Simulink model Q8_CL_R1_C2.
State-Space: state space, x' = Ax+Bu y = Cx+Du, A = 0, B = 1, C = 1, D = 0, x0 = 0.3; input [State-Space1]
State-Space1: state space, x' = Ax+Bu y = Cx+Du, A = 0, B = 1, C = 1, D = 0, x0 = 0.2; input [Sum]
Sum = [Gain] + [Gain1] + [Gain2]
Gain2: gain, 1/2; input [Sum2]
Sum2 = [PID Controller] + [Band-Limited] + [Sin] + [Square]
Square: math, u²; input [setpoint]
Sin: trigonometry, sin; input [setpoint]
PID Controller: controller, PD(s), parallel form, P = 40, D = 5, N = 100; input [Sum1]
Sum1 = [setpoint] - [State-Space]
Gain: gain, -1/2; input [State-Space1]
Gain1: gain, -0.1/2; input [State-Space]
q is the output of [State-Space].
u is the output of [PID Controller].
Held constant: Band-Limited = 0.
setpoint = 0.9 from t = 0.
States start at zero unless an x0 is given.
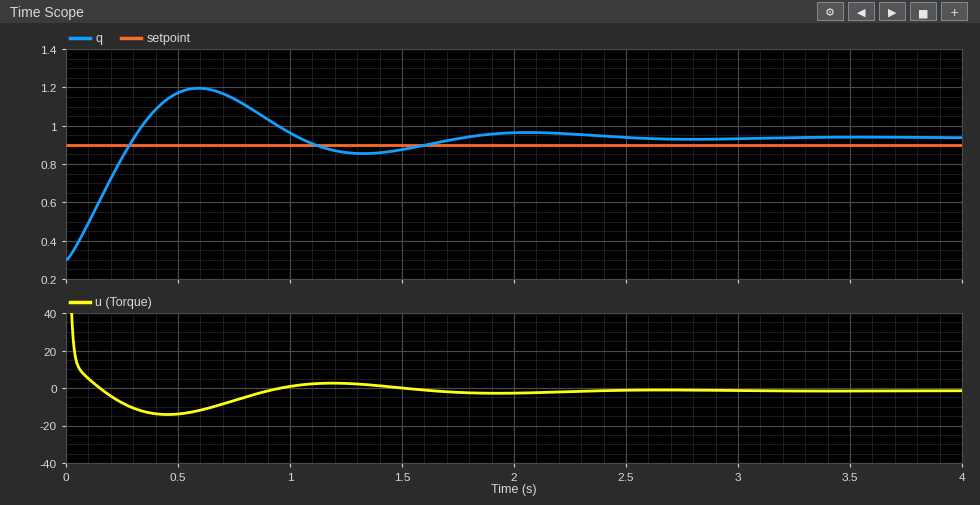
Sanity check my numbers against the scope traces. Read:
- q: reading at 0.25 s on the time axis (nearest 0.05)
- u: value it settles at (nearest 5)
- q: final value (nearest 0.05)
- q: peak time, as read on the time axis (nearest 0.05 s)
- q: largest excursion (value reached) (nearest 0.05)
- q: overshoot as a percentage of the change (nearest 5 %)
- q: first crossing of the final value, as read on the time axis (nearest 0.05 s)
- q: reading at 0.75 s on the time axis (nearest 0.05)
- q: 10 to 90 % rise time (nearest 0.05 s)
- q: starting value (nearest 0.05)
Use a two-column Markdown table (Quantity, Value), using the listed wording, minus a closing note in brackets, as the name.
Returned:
| Quantity | Value |
|---|---|
| q: reading at 0.25 s on the time axis | 0.85 |
| u: value it settles at | 0 |
| q: final value | 0.95 |
| q: peak time, as read on the time axis | 0.60 s |
| q: largest excursion (value reached) | 1.20 |
| q: overshoot as a percentage of the change | 40 % |
| q: first crossing of the final value, as read on the time axis | 0.30 s |
| q: reading at 0.75 s on the time axis | 1.15 |
| q: 10 to 90 % rise time | 0.25 s |
| q: starting value | 0.30 |
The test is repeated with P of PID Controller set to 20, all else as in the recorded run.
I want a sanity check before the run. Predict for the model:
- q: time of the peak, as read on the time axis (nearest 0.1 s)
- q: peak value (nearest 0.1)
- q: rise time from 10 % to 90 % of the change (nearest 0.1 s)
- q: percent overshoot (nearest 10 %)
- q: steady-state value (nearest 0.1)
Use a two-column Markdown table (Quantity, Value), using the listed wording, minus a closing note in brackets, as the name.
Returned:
| Quantity | Value |
|---|---|
| q: time of the peak, as read on the time axis | 0.8 s |
| q: peak value | 1.2 |
| q: rise time from 10 % to 90 % of the change | 0.3 s |
| q: percent overshoot | 30 % |
| q: steady-state value | 1.0 |
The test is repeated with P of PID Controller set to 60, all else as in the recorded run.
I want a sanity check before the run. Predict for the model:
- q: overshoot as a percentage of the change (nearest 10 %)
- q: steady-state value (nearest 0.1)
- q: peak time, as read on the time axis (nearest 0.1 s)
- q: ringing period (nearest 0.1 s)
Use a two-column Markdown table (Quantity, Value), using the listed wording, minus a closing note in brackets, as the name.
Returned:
| Quantity | Value |
|---|---|
| q: overshoot as a percentage of the change | 50 % |
| q: steady-state value | 0.9 |
| q: peak time, as read on the time axis | 0.5 s |
| q: ringing period | 1.2 s |
